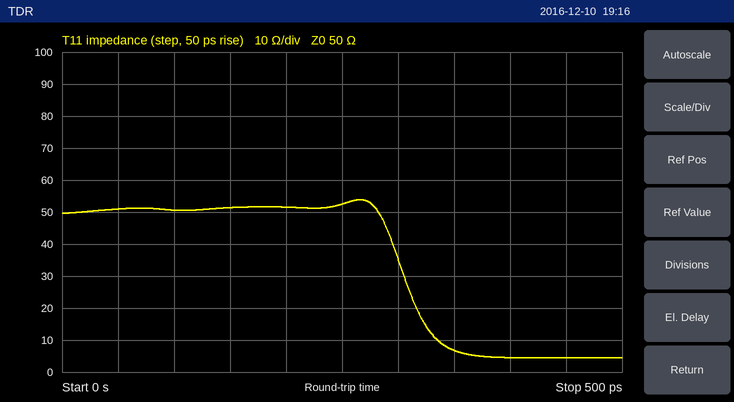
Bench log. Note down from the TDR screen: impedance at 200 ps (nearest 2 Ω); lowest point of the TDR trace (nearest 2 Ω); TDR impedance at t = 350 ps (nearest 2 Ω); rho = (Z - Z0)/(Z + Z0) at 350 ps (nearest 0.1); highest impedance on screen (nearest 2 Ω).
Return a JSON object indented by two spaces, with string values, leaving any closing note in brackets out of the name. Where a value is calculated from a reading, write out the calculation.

{
  "impedance at 200 ps": "52 Ω",
  "lowest point of the TDR trace": "4 Ω",
  "TDR impedance at t = 350 ps": "6 Ω",
  "rho = (Z - Z0)/(Z + Z0) at 350 ps": "(6 − 50)/(6 + 50) ≈ -0.8",
  "highest impedance on screen": "54 Ω"
}
